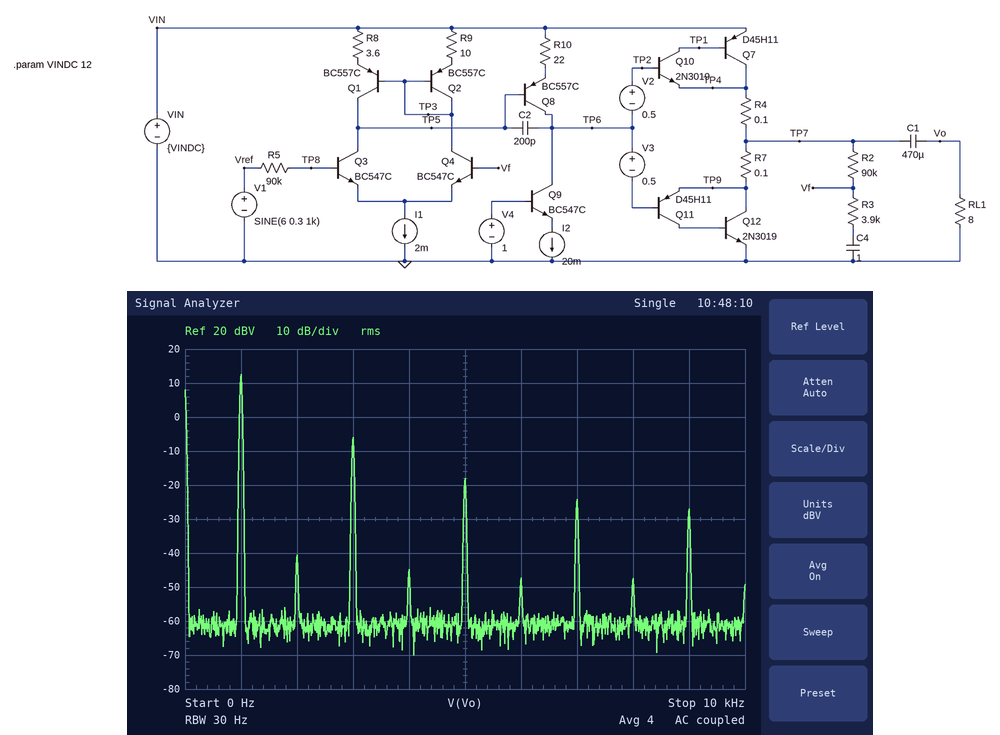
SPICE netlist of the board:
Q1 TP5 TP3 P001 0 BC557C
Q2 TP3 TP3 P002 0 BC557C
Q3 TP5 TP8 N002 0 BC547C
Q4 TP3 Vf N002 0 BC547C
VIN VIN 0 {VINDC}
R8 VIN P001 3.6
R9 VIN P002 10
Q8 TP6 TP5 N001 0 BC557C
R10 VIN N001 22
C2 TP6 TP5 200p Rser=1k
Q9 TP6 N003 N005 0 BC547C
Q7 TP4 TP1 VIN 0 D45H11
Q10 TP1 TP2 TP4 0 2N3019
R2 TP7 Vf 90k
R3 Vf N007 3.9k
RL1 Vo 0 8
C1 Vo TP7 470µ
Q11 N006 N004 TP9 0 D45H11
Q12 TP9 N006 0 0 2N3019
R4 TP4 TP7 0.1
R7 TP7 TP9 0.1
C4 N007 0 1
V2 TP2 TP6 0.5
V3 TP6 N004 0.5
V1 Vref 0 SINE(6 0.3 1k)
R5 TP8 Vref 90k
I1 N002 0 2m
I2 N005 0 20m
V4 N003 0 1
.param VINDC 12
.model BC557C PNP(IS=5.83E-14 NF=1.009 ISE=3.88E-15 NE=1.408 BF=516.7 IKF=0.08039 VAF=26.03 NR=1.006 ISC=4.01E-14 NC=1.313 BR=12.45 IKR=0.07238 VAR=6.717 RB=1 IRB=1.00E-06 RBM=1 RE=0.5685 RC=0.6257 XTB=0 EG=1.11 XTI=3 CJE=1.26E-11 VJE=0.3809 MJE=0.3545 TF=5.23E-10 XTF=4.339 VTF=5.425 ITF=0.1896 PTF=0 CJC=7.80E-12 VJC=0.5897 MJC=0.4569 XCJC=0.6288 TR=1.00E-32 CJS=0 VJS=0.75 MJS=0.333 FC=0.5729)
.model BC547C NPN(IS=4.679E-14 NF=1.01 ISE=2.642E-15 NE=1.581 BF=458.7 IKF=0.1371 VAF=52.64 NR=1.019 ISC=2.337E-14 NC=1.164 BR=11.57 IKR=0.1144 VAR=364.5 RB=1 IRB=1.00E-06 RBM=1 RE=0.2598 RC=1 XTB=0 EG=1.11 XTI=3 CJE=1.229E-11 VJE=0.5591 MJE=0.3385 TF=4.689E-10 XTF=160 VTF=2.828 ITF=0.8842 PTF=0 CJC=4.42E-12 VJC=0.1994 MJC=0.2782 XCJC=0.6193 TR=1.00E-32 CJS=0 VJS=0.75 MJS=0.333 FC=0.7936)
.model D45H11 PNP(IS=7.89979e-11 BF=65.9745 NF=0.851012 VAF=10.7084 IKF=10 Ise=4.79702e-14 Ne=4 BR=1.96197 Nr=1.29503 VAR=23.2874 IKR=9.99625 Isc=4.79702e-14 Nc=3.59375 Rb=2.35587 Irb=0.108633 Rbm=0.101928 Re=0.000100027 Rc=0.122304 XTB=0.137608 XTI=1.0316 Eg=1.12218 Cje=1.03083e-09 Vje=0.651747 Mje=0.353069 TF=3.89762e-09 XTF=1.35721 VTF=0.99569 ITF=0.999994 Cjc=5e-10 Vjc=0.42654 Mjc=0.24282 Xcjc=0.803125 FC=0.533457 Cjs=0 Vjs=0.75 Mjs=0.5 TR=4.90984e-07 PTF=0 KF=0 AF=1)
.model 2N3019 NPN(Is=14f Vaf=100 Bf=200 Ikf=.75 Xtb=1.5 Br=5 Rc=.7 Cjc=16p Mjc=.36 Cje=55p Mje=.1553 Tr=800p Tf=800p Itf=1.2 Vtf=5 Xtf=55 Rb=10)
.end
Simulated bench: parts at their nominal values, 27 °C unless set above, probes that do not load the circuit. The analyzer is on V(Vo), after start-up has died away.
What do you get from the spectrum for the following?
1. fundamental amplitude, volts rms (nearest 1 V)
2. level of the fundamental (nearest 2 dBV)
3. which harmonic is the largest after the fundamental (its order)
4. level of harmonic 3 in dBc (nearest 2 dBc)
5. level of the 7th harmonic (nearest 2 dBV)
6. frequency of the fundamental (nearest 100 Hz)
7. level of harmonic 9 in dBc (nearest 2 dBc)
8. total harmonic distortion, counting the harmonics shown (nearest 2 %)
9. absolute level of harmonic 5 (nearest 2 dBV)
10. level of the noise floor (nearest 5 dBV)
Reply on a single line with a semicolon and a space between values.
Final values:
4 V; 12 dBV; 3; -18 dBc; -24 dBV; 1.0 kHz; -40 dBc; 12 %; -18 dBV; -60 dBV
